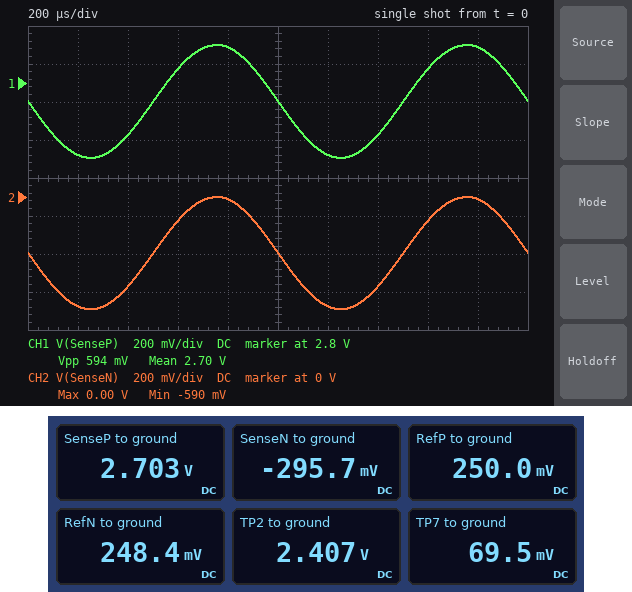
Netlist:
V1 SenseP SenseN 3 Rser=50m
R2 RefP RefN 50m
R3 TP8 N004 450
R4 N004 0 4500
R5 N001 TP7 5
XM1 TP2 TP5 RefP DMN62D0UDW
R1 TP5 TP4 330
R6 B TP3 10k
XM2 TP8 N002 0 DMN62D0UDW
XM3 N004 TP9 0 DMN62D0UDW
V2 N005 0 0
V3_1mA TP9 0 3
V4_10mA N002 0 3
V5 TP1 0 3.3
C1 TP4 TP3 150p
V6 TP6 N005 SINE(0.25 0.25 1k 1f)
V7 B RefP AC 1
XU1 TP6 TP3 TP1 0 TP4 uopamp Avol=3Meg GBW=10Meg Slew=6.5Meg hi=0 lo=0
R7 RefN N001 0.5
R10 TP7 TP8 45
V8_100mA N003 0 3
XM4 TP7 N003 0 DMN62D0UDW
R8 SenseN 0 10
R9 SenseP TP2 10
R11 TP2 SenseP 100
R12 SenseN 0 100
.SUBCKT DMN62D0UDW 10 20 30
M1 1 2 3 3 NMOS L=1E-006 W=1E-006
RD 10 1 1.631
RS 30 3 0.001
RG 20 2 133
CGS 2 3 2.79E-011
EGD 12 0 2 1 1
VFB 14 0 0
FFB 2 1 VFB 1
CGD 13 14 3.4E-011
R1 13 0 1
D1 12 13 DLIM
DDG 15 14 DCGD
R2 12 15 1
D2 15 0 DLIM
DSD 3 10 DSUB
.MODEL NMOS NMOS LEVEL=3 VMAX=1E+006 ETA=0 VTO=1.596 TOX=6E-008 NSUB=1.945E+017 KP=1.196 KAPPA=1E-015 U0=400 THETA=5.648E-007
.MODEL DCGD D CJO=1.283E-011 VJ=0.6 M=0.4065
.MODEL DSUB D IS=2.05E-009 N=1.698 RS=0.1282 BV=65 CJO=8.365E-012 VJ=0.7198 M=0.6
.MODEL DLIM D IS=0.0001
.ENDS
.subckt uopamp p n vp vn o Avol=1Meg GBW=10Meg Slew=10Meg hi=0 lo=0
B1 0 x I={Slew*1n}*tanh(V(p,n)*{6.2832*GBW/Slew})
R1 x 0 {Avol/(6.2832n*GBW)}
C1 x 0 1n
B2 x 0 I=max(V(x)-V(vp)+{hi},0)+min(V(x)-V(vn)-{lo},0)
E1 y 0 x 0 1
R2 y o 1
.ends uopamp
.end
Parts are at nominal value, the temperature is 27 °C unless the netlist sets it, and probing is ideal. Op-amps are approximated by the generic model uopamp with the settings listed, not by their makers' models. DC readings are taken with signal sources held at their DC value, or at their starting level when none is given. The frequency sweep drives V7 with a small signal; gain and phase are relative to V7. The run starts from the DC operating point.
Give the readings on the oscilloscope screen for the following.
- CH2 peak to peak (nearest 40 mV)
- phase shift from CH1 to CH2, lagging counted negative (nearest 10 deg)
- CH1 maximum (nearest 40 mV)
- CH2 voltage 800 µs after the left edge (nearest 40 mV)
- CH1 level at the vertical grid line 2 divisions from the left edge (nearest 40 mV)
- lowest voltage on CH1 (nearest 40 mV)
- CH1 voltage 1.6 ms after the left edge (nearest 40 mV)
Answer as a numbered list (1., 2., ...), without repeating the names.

1. 600 mV
2. 0 deg
3. 3.00 V
4. 0 V
5. 2.52 V
6. 2.40 V
7. 2.88 V
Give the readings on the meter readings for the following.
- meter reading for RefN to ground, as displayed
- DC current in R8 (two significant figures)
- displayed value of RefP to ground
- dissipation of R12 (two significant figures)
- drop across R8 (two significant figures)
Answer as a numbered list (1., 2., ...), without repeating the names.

1. 248.4 mV
2. 30 mA
3. 250.0 mV
4. 870 µW
5. 300 mV
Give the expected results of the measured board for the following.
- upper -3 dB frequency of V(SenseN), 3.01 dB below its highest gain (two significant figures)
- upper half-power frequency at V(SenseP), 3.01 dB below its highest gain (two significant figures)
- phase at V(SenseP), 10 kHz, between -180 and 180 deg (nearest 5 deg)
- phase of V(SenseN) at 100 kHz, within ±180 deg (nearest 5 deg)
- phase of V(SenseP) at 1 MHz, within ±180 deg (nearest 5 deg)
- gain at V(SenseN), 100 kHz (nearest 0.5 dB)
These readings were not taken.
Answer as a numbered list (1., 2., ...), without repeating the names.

1. 63 kHz
2. 63 kHz
3. -10 deg
4. -60 deg
5. -100 deg
6. -4.0 dB
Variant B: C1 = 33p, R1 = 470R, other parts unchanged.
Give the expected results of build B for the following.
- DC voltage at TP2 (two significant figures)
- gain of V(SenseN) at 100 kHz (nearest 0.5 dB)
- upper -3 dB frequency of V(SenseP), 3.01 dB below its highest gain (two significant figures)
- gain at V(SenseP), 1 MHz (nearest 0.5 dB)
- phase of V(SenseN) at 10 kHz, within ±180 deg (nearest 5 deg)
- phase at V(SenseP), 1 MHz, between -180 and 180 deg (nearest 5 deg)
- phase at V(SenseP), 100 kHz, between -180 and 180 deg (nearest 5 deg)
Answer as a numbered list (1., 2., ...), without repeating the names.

1. 2.4 V
2. 1.0 dB
3. 290 kHz
4. -9.5 dB
5. 0 deg
6. -90 deg
7. -20 deg
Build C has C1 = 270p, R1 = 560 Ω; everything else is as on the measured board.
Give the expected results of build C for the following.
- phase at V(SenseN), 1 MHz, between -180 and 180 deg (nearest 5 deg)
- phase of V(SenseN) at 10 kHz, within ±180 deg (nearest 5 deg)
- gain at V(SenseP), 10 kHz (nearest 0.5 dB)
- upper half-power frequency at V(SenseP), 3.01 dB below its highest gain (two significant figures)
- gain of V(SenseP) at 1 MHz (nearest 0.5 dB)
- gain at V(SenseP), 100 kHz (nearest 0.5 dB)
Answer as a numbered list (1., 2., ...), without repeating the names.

1. -105 deg
2. -15 deg
3. 1.0 dB
4. 35 kHz
5. -28.0 dB
6. -8.0 dB
